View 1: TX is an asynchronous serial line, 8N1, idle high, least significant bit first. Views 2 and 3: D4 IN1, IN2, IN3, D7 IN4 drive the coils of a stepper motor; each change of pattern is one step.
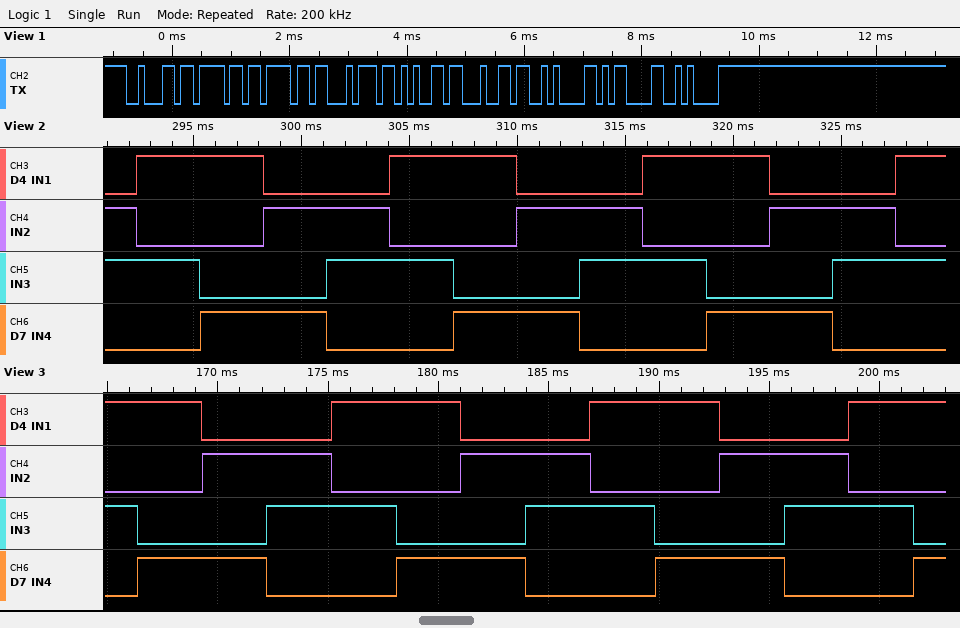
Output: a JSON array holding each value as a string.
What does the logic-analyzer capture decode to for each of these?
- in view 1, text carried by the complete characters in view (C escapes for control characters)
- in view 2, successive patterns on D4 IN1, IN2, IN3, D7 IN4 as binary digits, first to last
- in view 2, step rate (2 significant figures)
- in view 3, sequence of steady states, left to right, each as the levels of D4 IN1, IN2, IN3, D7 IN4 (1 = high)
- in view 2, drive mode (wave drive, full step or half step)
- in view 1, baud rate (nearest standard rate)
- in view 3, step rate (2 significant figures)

["\"booted\\n\\r\\n\"", "0110 1010 1001 0101 0110 1010 1001 0101 0110 1010 1001 0101 0110 1010", "340 steps/s", "1010 1001 0101 0110 1010 1001 0101 0110 1010 1001 0101 0110 1010 1001", "full step", "9600 baud", "340 steps/s"]
